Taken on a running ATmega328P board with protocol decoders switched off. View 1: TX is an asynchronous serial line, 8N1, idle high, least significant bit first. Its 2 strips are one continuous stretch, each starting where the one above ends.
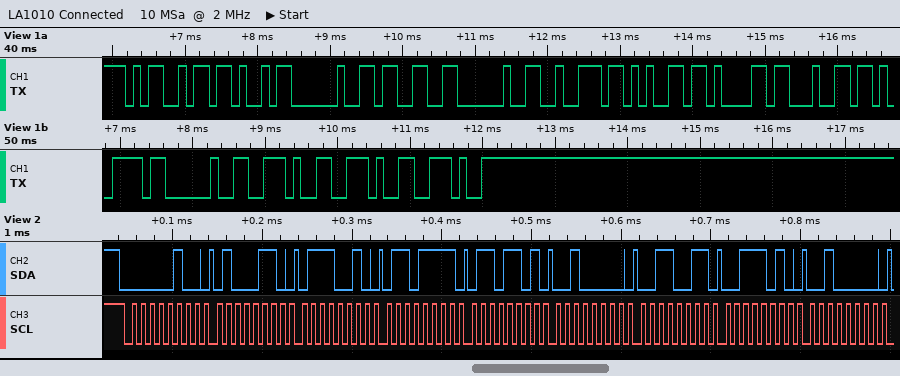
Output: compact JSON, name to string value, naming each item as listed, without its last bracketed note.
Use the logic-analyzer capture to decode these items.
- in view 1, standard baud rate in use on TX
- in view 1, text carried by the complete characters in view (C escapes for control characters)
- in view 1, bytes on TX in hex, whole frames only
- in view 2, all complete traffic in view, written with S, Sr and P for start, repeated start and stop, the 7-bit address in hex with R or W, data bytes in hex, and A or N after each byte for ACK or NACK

{"in view 1, standard baud rate in use on TX": "9600 baud", "in view 1, text carried by the complete characters in view": "\"MK 3 ready ...\"", "in view 1, bytes on TX in hex, whole frames only": "0x4D 0x4B 0x20 0x33 0x20 0x72 0x65 0x61 0x64 0x79 0x20 0x2E 0x2E 0x2E", "in view 2, all complete traffic in view, written with S, Sr and P for start, repeated start and stop, the 7-bit address in hex with R or W, data bytes in hex, and A or N after each byte for ACK or NACK": "S 02W A 46 A 72 A 6F A 6D A 20 A 33 A 3A A 20 A"}
